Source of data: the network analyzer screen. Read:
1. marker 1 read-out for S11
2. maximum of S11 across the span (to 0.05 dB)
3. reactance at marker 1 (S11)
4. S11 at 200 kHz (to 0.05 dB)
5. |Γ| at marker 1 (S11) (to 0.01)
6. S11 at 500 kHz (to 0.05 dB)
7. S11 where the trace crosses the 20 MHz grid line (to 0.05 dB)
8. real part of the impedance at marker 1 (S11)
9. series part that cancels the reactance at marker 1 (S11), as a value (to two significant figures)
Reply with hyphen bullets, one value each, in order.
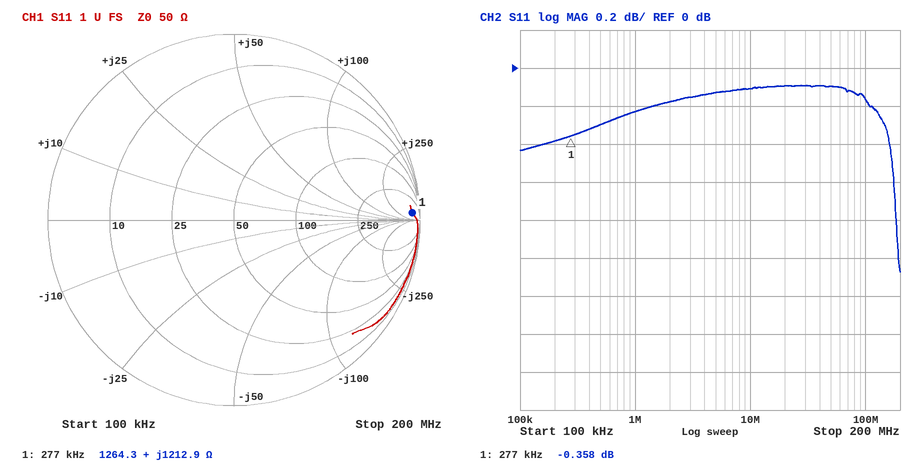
- -0.358 dB
- -0.10 dB
- +1212.9 Ω
- -0.40 dB
- 0.96
- -0.30 dB
- -0.10 dB
- 1264.3 Ω
- 470 pF
